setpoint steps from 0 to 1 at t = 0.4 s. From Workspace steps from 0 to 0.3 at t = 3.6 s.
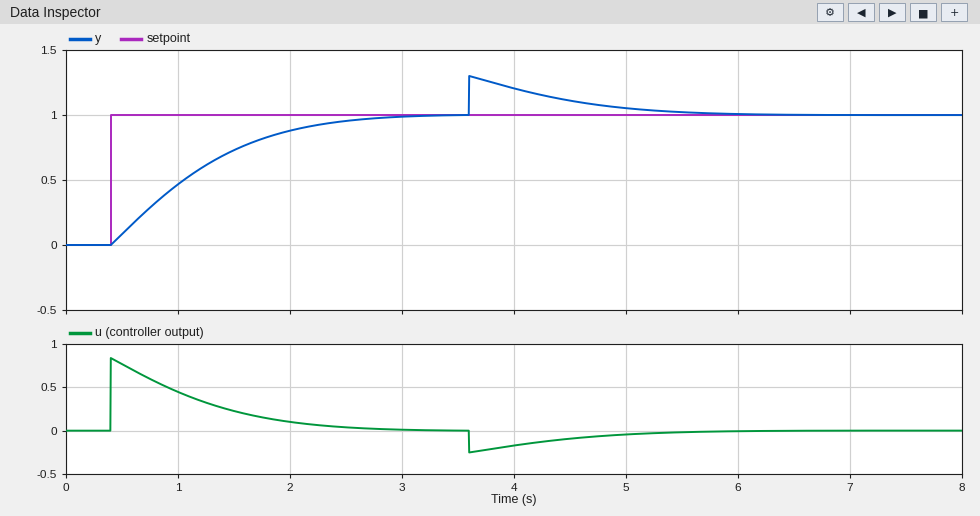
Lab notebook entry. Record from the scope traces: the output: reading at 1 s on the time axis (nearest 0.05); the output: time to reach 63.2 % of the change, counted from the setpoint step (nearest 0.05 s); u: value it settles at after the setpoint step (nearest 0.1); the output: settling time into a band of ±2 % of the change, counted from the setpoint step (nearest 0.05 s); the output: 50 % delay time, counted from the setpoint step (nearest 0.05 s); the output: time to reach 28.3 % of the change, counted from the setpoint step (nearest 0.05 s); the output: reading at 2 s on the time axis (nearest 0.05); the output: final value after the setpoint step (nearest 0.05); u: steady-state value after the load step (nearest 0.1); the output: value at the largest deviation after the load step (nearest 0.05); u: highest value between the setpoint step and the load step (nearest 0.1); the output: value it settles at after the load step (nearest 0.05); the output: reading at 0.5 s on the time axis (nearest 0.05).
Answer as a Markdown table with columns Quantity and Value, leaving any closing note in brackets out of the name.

| Quantity | Value |
|---|---|
| the output: reading at 1 s on the time axis | 0.45 |
| the output: time to reach 63.2 % of the change, counted from the setpoint step | 0.90 s |
| u: value it settles at after the setpoint step | 0.0 |
| the output: settling time into a band of ±2 % of the change, counted from the setpoint step | 2.45 s |
| the output: 50 % delay time, counted from the setpoint step | 0.65 s |
| the output: time to reach 28.3 % of the change, counted from the setpoint step | 0.35 s |
| the output: reading at 2 s on the time axis | 0.90 |
| the output: final value after the setpoint step | 1.00 |
| u: steady-state value after the load step | 0.0 |
| the output: value at the largest deviation after the load step | 1.30 |
| u: highest value between the setpoint step and the load step | 0.8 |
| the output: value it settles at after the load step | 1.00 |
| the output: reading at 0.5 s on the time axis | 0.10 |
